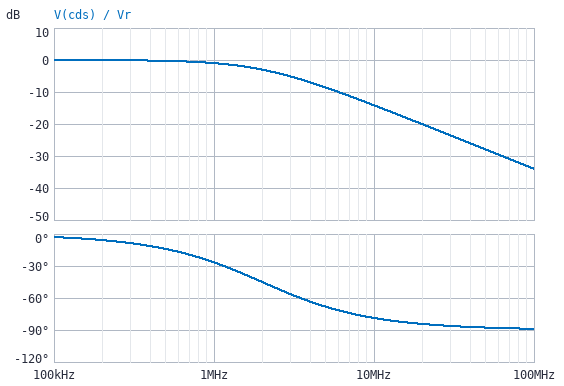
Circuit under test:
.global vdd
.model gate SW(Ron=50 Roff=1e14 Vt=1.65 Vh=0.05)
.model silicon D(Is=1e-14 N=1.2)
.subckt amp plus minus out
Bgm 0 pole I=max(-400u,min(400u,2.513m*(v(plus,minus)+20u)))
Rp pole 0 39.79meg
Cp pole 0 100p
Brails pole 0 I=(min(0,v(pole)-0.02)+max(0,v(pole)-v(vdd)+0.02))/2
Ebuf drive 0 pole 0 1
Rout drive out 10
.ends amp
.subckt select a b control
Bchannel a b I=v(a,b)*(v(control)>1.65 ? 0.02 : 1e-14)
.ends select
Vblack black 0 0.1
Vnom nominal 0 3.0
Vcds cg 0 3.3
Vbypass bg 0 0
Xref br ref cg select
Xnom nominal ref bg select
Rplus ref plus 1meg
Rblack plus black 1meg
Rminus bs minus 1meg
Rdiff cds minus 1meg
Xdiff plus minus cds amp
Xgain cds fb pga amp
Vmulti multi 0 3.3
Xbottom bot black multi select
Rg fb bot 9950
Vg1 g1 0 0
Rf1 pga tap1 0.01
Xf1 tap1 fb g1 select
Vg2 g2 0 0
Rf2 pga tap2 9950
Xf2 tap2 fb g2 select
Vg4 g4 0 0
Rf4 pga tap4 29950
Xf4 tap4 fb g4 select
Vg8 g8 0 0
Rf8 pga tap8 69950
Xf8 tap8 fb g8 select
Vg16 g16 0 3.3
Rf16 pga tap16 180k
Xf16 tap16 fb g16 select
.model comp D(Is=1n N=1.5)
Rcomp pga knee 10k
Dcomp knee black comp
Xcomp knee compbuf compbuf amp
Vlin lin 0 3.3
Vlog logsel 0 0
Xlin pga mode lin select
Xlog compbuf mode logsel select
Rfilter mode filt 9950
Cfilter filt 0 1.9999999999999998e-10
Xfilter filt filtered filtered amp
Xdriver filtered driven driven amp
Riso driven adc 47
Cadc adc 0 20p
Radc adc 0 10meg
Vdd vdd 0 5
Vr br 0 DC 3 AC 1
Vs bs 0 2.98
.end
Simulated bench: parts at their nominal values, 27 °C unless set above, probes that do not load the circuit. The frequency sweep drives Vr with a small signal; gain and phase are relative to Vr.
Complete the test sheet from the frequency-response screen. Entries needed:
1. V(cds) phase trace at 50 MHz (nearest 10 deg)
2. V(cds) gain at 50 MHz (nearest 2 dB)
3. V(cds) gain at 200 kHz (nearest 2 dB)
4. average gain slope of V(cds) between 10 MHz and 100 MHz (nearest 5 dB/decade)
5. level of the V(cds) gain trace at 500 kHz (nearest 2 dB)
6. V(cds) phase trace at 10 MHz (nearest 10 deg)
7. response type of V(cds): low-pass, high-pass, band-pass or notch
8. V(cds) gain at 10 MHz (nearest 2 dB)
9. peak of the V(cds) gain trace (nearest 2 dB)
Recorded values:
-90 deg
-28 dB
0 dB
-20 dB/decade
0 dB
-80 deg
low-pass
-14 dB
0 dB
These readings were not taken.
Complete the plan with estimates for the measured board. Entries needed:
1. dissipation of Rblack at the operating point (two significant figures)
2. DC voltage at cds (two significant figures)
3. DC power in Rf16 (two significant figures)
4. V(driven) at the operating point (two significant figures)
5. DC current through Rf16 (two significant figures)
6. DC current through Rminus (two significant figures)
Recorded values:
2.1 µW
120 mV
720 nW
480 mV
2.0 µA
1.4 µA
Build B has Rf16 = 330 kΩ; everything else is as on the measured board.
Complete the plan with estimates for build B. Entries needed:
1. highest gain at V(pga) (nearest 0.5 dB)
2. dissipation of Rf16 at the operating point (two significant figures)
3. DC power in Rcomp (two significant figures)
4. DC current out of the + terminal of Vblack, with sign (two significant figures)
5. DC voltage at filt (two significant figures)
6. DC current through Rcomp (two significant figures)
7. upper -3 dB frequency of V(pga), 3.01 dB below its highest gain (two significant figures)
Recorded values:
30.5 dB
1.3 µW
7.9 µW
-32 µA
780 mV
28 µA
120 kHz
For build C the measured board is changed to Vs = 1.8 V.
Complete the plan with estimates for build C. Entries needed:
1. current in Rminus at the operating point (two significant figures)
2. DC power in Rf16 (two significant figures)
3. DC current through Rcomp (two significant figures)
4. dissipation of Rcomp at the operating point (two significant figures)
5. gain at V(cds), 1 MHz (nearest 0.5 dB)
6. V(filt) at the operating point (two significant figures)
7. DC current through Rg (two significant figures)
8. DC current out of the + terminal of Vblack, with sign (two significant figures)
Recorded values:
250 nA
120 µW
440 µA
1.9 mW
-1.0 dB
5.0 V
26 µA
-460 µA
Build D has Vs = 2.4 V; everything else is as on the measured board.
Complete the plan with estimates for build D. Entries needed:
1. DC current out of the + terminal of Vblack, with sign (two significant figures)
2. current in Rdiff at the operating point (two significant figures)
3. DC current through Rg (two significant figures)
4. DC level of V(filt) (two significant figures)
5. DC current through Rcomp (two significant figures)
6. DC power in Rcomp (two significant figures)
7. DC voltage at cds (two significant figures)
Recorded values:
-460 µA
850 nA
26 µA
5.0 V
440 µA
1.9 mW
700 mV
